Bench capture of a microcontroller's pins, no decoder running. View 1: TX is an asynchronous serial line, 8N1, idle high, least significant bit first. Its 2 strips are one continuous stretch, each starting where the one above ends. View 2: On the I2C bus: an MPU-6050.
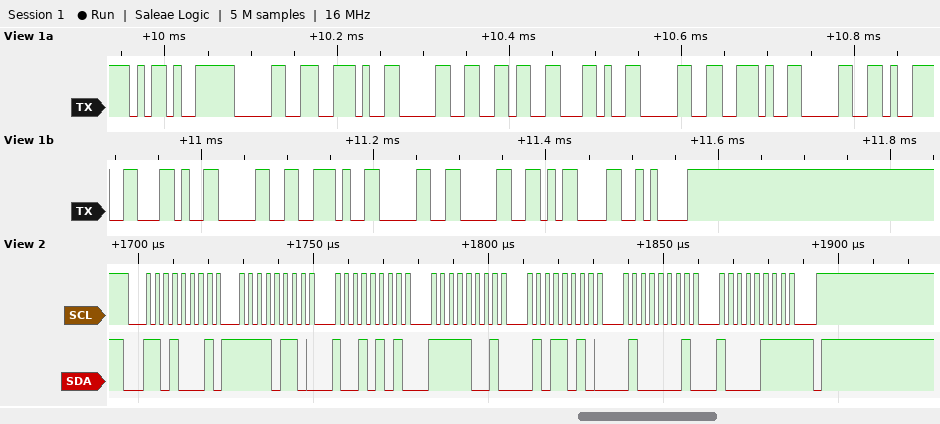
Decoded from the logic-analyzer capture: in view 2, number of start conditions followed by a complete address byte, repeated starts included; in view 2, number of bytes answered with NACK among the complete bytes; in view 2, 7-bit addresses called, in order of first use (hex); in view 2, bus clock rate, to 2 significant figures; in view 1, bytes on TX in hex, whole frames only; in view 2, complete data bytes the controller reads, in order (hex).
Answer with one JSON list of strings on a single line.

["1", "1", "0x68", "400 kHz", "0x2D 0x30 0x2E 0x30 0x36 0x2C 0x30 0x2E 0x30 0x39 0x2C 0x30 0x2E 0x30 0x30 0x0D 0x0A", "F6 95 F9 5A 41 87"]
